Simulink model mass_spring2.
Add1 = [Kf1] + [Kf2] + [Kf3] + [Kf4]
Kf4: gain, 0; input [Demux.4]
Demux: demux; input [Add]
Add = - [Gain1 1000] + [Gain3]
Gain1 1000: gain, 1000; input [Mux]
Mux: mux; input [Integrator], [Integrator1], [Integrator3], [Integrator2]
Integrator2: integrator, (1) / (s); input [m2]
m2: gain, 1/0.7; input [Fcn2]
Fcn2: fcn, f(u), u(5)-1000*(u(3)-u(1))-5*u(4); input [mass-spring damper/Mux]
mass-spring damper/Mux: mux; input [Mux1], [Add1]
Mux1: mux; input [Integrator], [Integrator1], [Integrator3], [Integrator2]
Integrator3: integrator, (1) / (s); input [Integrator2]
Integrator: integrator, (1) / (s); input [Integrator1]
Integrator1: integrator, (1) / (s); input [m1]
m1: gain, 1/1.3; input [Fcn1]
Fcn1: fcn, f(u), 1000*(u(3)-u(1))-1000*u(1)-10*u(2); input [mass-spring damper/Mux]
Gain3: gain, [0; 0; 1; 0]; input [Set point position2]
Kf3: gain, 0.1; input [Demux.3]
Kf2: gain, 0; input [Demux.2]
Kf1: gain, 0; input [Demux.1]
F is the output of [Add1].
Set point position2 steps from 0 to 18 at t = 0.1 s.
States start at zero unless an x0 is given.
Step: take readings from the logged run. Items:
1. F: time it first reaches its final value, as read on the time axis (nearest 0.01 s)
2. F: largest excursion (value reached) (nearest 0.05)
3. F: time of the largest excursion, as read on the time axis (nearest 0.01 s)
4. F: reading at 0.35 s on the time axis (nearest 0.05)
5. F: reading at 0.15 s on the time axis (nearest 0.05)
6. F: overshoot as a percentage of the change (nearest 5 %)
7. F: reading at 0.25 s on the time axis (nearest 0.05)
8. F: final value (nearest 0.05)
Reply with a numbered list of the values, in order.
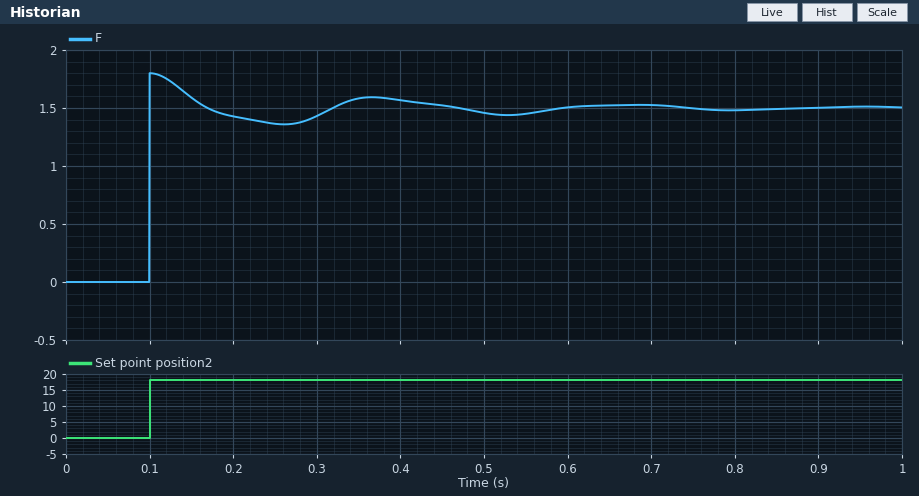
1. 0.10 s
2. 1.80
3. 0.10 s
4. 1.60
5. 1.60
6. 20 %
7. 1.35
8. 1.50
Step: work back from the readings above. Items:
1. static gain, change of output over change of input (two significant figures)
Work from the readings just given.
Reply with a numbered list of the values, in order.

1. 0.083
